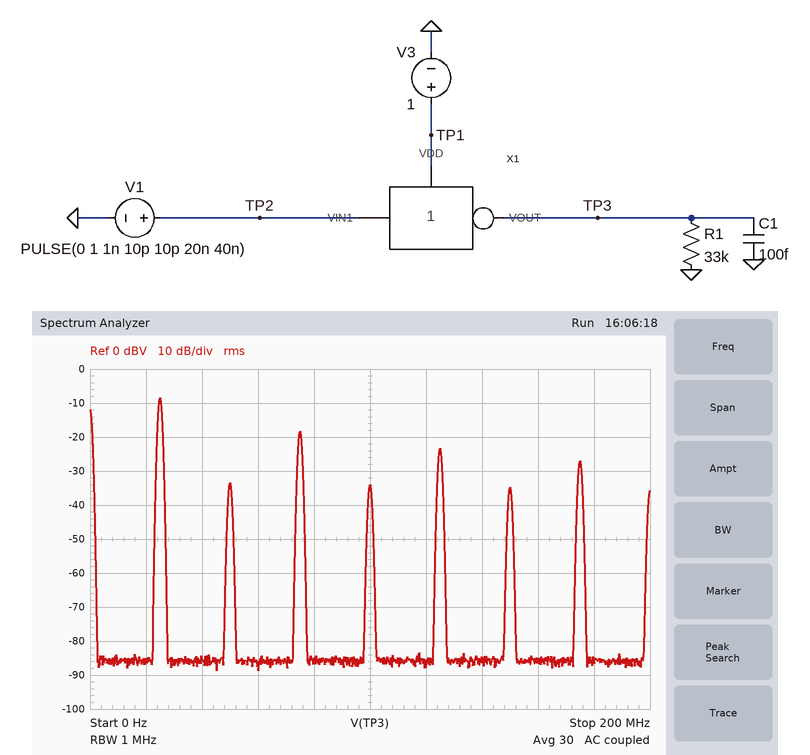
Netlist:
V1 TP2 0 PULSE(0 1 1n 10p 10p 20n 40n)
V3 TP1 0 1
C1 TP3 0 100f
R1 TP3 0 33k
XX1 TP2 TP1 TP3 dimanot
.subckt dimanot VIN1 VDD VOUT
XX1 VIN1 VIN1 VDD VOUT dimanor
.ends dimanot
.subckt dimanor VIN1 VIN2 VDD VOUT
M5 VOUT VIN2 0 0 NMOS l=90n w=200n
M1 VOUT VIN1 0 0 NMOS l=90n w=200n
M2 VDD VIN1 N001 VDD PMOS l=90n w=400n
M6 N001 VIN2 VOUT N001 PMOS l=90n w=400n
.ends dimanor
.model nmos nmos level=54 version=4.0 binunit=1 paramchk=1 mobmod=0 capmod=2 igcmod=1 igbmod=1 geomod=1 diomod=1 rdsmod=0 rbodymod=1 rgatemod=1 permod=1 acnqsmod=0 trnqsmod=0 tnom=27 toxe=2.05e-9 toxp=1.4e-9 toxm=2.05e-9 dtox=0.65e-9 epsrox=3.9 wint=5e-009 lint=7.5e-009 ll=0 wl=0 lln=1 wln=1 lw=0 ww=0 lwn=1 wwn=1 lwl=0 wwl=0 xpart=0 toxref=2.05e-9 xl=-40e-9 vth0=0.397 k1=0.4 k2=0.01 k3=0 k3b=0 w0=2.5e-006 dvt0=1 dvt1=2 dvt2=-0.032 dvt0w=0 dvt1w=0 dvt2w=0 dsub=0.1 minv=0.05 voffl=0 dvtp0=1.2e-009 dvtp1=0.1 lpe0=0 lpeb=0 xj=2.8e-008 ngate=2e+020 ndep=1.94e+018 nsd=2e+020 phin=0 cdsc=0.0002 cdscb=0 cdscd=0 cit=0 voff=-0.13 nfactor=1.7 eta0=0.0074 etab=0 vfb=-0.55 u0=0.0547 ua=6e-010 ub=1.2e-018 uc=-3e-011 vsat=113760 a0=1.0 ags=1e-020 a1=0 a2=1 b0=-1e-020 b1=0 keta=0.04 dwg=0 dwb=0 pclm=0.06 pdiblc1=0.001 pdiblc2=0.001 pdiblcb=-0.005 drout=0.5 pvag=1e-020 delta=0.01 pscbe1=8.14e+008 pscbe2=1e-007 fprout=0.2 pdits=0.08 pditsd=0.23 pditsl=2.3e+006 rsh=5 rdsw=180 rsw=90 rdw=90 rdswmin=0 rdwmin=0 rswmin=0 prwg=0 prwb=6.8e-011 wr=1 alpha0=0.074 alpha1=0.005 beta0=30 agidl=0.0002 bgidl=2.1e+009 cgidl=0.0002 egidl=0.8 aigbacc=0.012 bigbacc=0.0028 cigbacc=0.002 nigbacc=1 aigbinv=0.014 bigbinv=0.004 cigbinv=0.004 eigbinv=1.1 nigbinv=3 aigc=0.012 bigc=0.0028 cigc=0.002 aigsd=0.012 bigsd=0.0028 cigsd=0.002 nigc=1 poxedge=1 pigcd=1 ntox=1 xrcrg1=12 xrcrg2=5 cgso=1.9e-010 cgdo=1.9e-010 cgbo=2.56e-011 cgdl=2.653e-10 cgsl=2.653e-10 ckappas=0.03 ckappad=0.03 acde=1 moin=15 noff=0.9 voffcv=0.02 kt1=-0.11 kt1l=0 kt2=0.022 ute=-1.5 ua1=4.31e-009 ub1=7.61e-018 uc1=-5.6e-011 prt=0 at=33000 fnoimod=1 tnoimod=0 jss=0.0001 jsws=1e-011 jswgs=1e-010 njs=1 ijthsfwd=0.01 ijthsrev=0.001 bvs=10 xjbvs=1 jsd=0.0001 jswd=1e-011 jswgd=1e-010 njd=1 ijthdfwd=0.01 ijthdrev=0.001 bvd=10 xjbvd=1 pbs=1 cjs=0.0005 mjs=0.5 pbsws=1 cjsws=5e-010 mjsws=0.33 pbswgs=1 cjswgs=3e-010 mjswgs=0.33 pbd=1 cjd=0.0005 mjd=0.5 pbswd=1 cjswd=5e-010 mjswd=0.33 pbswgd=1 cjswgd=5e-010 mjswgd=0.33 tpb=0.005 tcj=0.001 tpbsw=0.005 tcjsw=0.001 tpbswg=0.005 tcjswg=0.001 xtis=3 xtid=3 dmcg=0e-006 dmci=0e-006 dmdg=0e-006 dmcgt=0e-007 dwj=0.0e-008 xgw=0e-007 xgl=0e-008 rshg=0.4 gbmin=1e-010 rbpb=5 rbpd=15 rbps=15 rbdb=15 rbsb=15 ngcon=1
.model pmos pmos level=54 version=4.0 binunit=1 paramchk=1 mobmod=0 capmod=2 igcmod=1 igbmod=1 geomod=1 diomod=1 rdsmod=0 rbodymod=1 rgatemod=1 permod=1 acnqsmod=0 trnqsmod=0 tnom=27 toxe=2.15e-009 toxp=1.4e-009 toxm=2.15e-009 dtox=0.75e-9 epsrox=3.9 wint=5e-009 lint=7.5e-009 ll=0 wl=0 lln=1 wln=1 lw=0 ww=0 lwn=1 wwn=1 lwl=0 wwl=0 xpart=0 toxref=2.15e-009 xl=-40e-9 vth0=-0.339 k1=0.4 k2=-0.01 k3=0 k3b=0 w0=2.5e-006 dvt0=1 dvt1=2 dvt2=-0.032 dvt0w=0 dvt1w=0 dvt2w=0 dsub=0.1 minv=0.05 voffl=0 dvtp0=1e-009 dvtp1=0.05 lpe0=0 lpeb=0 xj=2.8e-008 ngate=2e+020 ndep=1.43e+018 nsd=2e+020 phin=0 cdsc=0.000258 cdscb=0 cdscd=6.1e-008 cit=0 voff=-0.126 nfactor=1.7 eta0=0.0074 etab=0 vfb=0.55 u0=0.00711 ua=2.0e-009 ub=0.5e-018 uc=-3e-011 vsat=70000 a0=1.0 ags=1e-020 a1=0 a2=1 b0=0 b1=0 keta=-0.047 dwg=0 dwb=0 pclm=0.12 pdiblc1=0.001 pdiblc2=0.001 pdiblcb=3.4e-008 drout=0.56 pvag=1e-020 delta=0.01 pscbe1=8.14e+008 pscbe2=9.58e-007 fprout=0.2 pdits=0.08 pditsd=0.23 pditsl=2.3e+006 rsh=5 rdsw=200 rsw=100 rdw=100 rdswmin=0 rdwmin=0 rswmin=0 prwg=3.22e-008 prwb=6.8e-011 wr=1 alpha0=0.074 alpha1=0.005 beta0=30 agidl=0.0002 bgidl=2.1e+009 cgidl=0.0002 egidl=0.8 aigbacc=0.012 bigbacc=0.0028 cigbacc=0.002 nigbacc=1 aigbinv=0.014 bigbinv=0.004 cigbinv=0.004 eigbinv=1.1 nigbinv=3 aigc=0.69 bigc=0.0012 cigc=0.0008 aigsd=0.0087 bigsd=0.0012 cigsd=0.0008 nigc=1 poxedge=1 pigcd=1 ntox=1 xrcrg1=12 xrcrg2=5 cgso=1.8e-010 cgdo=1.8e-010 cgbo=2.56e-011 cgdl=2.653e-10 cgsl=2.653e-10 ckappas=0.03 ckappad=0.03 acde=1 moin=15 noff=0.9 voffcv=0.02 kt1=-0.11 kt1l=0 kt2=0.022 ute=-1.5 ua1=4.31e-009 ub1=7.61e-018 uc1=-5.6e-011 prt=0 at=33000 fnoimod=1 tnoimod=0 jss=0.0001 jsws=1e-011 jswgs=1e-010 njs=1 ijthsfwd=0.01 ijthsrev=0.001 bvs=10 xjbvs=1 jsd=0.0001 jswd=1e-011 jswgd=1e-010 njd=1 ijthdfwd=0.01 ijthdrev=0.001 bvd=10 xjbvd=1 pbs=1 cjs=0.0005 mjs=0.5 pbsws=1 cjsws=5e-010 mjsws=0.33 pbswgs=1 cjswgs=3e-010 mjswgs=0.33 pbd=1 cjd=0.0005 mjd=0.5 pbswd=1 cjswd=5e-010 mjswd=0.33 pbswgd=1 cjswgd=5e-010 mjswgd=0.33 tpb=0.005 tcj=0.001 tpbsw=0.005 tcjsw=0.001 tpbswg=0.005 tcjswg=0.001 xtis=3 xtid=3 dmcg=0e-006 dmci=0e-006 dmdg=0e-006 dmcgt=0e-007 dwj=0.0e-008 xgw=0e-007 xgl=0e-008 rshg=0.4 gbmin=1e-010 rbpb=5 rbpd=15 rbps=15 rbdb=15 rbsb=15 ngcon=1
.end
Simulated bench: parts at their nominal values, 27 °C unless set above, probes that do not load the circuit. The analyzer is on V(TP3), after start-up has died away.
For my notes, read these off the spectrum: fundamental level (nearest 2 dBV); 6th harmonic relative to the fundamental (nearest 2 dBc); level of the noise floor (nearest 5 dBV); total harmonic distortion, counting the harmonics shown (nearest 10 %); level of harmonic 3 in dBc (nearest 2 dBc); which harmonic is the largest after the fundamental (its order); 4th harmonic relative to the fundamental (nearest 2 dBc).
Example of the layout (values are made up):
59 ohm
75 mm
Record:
-8 dBV
-26 dBc
-85 dBV
40 %
-10 dBc
3
-26 dBc
